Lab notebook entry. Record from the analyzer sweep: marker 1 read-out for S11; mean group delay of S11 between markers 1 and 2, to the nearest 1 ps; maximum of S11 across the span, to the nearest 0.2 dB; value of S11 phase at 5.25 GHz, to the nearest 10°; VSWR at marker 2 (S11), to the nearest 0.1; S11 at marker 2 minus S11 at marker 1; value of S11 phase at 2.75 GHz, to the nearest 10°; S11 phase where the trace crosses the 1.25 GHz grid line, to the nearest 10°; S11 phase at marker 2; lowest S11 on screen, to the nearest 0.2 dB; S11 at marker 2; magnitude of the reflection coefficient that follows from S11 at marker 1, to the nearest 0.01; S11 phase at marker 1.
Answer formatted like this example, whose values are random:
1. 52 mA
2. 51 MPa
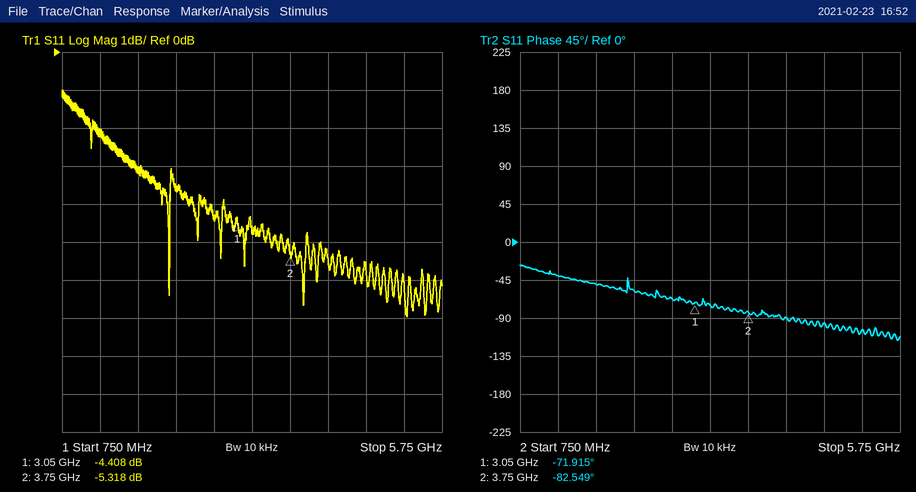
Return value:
1. -4.408 dB
2. 42 ps
3. -1.0 dB
4. -100°
5. 3.4
6. -0.910 dB
7. -70°
8. -40°
9. -82.549°
10. -7.0 dB
11. -5.318 dB
12. 0.60
13. -71.915°
